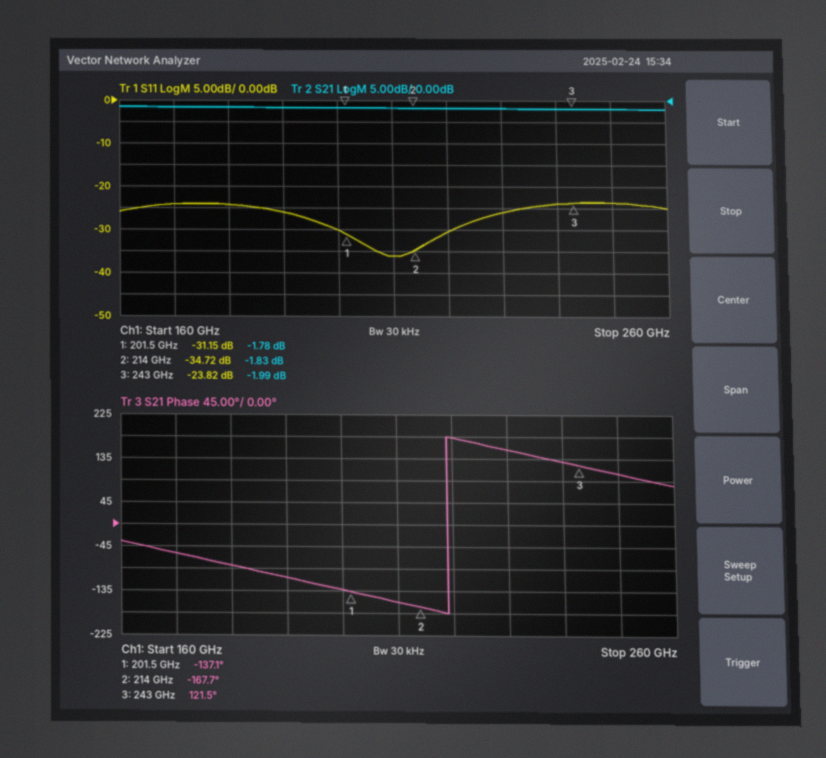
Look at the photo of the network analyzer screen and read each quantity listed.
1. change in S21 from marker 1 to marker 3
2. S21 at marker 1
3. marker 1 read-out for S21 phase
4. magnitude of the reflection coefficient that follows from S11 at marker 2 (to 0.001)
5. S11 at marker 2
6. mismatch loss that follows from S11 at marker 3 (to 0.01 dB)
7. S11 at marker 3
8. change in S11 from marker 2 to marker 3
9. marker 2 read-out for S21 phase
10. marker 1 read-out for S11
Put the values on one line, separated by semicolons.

-0.21 dB; -1.78 dB; -137.1°; 0.018; -34.72 dB; 0.02 dB; -23.82 dB; 10.90 dB; -167.7°; -31.15 dB
